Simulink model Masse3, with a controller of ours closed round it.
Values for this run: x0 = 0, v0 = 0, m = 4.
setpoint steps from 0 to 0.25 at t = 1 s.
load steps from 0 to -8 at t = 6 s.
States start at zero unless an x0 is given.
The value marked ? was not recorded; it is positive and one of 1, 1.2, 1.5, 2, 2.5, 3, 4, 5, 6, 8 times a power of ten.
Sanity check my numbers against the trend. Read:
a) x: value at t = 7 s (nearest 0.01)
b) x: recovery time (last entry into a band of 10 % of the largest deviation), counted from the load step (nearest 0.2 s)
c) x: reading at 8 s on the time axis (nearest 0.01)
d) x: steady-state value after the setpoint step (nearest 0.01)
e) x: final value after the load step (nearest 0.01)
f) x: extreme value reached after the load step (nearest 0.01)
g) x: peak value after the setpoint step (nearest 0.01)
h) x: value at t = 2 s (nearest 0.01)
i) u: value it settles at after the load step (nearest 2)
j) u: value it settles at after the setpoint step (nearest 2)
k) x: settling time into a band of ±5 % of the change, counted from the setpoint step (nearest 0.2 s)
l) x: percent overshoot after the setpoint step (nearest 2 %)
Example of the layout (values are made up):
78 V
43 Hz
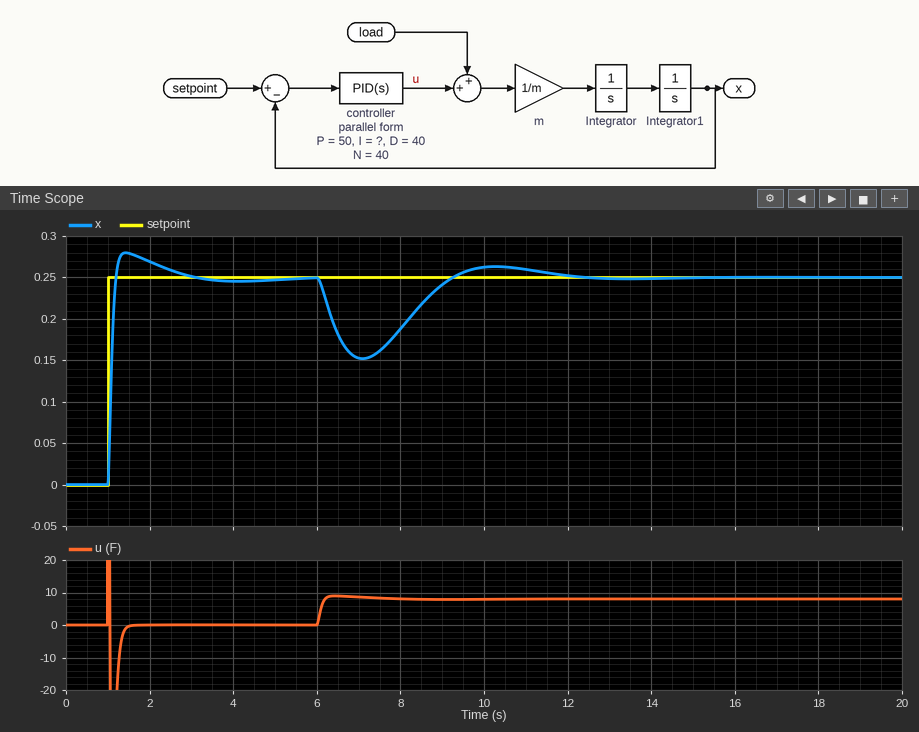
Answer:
0.15
5.0 s
0.19
0.25
0.25
0.15
0.28
0.27
8
0
1.4 s
12 %
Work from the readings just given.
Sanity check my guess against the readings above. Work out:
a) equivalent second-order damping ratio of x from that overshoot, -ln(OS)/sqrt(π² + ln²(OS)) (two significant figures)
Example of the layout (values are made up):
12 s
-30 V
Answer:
0.56
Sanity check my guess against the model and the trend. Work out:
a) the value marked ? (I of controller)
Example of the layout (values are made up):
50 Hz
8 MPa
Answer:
50
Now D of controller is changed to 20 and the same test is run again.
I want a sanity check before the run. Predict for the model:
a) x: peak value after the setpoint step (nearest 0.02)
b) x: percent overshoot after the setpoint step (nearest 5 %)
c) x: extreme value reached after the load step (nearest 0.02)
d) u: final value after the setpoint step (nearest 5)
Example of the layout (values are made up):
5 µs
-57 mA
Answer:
0.32
30 %
0.12
0
